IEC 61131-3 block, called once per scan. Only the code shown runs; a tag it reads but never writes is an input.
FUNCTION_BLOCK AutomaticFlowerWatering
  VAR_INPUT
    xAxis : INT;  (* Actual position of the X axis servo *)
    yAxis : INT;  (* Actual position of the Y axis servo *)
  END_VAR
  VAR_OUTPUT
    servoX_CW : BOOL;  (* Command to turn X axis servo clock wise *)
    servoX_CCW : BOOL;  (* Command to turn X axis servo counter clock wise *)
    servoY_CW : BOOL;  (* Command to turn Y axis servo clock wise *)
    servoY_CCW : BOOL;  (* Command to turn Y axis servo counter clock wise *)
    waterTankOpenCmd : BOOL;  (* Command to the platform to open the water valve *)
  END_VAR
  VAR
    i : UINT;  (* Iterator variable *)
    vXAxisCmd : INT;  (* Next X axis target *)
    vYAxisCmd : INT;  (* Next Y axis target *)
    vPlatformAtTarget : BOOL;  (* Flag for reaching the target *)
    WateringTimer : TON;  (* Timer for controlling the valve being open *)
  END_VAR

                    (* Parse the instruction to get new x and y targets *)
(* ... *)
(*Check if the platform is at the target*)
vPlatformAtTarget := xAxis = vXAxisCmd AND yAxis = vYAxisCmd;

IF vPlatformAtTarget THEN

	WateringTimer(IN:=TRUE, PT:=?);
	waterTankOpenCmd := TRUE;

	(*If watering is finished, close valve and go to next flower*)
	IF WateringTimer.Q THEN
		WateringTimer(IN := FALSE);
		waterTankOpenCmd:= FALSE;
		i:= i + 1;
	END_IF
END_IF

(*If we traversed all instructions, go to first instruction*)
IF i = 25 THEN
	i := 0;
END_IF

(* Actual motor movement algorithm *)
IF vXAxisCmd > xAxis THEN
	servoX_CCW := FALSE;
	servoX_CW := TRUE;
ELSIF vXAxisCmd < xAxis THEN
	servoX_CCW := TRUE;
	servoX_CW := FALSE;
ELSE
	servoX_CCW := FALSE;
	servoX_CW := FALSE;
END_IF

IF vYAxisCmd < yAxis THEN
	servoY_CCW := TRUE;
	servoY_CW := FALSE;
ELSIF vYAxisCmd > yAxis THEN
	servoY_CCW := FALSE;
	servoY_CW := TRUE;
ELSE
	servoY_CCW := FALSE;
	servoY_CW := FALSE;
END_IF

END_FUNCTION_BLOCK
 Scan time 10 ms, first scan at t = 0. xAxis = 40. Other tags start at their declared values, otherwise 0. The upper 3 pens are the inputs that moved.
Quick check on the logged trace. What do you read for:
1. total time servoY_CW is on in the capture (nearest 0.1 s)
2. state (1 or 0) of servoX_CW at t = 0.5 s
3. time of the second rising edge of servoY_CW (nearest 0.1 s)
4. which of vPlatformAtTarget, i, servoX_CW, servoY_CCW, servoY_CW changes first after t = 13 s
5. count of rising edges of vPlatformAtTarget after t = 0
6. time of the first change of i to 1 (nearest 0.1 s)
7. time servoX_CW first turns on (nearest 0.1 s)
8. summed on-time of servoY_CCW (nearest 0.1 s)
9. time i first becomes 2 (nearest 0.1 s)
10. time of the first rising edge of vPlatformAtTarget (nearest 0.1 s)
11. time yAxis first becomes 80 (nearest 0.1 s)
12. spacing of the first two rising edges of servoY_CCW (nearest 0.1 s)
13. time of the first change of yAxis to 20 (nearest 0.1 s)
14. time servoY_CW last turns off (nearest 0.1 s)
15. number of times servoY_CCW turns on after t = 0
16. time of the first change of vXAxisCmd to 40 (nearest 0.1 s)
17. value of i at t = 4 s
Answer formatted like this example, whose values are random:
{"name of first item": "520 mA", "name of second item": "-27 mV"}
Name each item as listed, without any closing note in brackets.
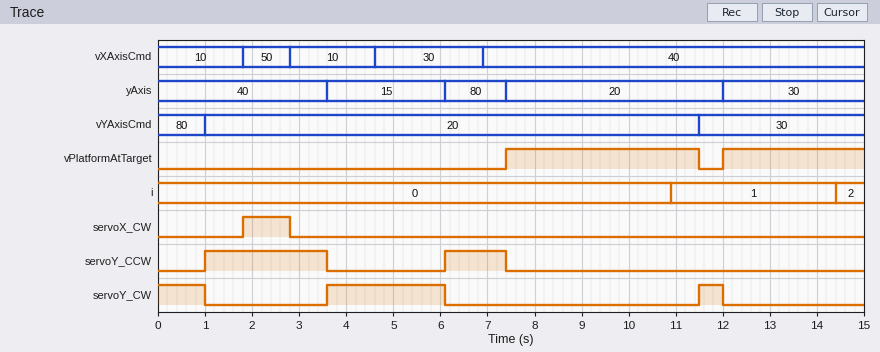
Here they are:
{"total time servoY_CW is on in the capture": "4.0 s", "state (1 or 0) of servoX_CW at t = 0.5 s": "0", "time of the second rising edge of servoY_CW": "11.5 s", "which of vPlatformAtTarget, i, servoX_CW, servoY_CCW, servoY_CW changes first after t = 13 s": "i", "count of rising edges of vPlatformAtTarget after t = 0": "2", "time of the first change of i to 1": "10.9 s", "time servoX_CW first turns on": "1.8 s", "summed on-time of servoY_CCW": "3.9 s", "time i first becomes 2": "14.4 s", "time of the first rising edge of vPlatformAtTarget": "7.4 s", "time yAxis first becomes 80": "6.1 s", "spacing of the first two rising edges of servoY_CCW": "5.1 s", "time of the first change of yAxis to 20": "7.4 s", "time servoY_CW last turns off": "12.0 s", "number of times servoY_CCW turns on after t = 0": "2", "time of the first change of vXAxisCmd to 40": "6.9 s", "value of i at t = 4 s": "0"}
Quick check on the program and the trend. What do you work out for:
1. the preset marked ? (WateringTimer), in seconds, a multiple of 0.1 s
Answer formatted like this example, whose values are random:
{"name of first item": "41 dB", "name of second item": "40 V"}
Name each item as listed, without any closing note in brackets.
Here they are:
{"the preset marked ? (WateringTimer), in seconds, a multiple of 0.1 s": "3.5 s"}
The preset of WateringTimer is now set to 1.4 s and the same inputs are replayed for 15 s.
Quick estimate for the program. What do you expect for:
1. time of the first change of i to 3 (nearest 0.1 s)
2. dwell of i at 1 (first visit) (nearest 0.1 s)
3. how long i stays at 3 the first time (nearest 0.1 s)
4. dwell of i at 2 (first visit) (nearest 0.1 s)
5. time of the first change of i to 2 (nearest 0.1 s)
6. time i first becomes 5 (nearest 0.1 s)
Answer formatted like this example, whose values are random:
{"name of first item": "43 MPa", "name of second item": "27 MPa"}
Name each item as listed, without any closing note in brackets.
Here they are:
{"time of the first change of i to 3": "12.0 s", "dwell of i at 1 (first visit)": "1.4 s", "how long i stays at 3 the first time": "1.4 s", "dwell of i at 2 (first visit)": "1.8 s", "time of the first change of i to 2": "10.2 s", "time i first becomes 5": "14.8 s"}
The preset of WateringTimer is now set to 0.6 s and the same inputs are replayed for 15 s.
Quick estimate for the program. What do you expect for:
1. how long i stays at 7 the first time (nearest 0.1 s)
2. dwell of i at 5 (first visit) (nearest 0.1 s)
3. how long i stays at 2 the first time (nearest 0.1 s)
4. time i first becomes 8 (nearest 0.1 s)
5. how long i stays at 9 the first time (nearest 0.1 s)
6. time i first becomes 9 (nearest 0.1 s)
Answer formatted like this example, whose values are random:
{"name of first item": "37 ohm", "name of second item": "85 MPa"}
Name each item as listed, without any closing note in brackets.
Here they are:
{"how long i stays at 7 the first time": "0.6 s", "dwell of i at 5 (first visit)": "0.6 s", "how long i stays at 2 the first time": "0.6 s", "time i first becomes 8": "12.6 s", "how long i stays at 9 the first time": "0.6 s", "time i first becomes 9": "13.2 s"}
